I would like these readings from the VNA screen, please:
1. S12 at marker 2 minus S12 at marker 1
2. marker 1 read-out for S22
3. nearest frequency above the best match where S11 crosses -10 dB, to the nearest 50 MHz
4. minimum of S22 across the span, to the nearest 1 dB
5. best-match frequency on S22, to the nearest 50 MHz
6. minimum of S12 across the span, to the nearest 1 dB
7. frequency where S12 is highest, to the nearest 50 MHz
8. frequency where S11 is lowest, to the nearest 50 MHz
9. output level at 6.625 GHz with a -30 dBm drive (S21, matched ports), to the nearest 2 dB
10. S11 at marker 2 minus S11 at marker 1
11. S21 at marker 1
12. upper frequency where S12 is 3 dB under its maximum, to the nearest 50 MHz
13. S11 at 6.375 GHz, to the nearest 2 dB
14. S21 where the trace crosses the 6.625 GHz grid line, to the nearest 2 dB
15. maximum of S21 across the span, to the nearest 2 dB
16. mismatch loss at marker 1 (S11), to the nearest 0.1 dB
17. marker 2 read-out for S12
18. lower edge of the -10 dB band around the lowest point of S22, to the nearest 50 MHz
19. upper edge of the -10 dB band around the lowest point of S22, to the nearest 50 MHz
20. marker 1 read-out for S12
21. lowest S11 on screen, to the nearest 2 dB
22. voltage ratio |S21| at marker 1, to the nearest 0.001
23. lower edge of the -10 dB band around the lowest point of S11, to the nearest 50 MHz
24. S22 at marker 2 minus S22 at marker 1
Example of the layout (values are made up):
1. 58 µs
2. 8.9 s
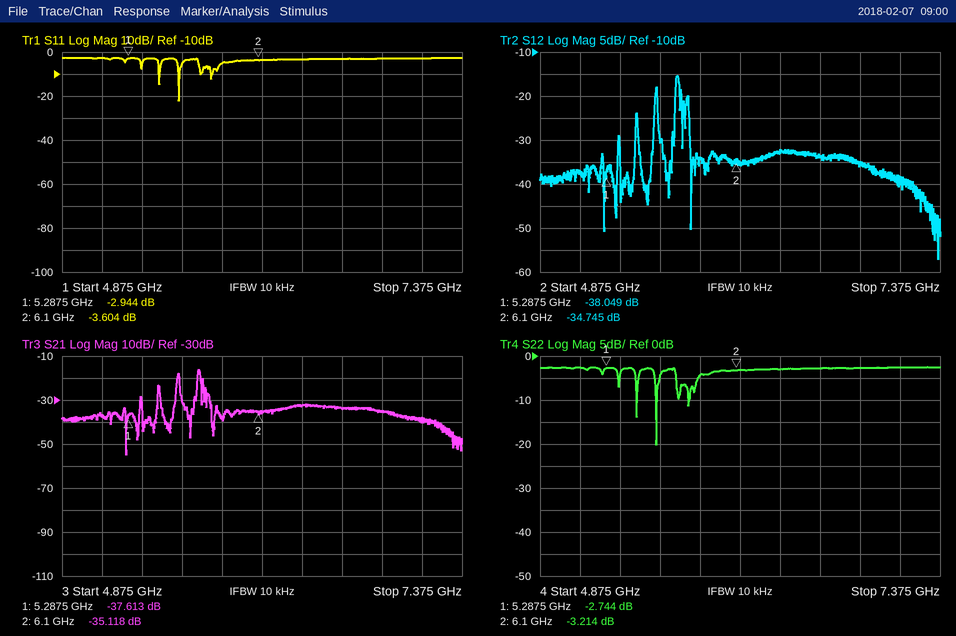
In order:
1. 3.304 dB
2. -2.744 dB
3. 5.60 GHz
4. -20 dB
5. 5.60 GHz
6. -57 dB
7. 5.75 GHz
8. 5.60 GHz
9. -64 dBm
10. -0.660 dB
11. -37.613 dB
12. 5.75 GHz
13. -4 dB
14. -34 dB
15. -16 dB
16. 3.1 dB
17. -34.745 dB
18. 5.60 GHz
19. 5.60 GHz
20. -38.049 dB
21. -22 dB
22. 0.013
23. 5.60 GHz
24. -0.470 dB
